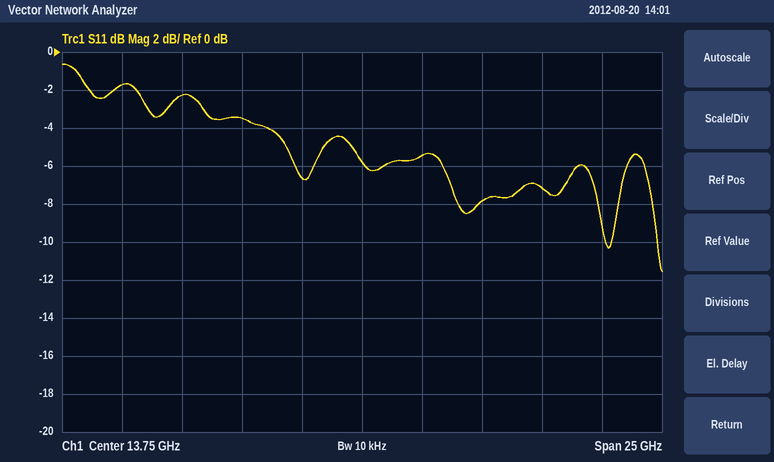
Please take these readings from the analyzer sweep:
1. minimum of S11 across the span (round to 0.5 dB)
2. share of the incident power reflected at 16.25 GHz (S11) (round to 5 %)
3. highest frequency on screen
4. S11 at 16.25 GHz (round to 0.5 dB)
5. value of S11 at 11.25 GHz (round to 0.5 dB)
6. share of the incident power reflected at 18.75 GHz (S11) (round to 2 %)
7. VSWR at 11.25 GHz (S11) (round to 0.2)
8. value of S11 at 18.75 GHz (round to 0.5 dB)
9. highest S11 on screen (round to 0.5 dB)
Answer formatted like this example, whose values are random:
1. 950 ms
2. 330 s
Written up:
1. -11.5 dB
2. 30 %
3. 26.25 GHz
4. -5.5 dB
5. -6.5 dB
6. 16 %
7. 2.8
8. -8.0 dB
9. -0.5 dB
